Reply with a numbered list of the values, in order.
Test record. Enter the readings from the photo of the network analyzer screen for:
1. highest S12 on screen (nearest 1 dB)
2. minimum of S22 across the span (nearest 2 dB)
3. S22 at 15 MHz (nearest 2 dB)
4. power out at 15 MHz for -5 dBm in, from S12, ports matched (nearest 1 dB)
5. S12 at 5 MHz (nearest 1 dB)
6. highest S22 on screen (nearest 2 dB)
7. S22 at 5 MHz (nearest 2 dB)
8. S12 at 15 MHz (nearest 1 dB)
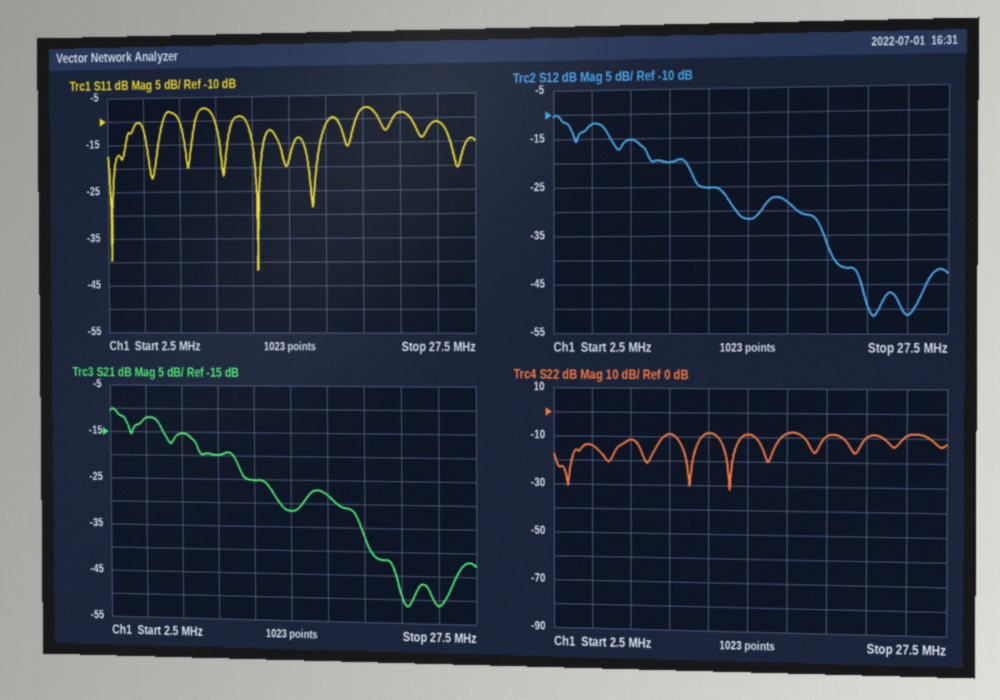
1. -10 dB
2. -32 dB
3. -8 dB
4. -37 dBm
5. -12 dB
6. -8 dB
7. -14 dB
8. -32 dB
